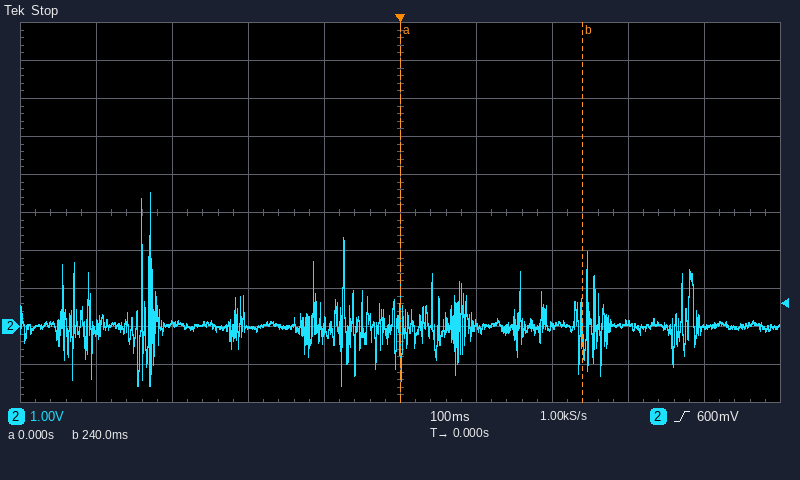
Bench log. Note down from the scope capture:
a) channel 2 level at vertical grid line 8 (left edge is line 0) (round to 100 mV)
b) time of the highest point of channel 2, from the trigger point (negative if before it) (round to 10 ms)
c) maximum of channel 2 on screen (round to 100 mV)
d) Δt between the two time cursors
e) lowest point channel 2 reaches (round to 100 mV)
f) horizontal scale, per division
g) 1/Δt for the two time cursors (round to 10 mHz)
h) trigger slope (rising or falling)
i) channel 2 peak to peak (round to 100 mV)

100 mV
-330 ms
3.5 V
240 ms
-1.6 V
100 ms
4.17 Hz
rising
5.1 V
